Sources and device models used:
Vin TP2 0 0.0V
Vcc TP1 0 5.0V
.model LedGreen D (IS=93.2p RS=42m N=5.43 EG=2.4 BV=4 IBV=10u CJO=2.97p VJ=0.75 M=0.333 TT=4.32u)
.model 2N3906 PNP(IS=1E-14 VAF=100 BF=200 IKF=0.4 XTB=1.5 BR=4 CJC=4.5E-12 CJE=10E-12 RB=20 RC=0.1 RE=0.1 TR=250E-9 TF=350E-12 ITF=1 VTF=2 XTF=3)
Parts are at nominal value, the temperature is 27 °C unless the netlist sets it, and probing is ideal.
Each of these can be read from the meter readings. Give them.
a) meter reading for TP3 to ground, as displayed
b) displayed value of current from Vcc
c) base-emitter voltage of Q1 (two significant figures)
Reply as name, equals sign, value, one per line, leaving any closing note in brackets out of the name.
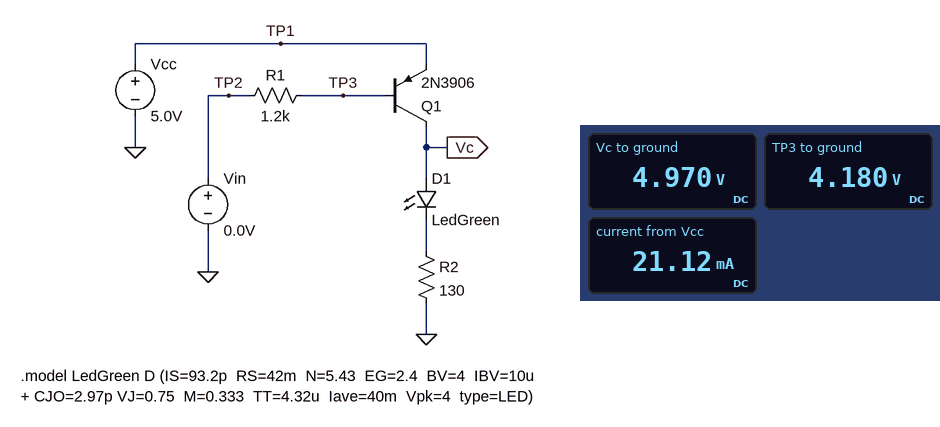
meter reading for TP3 to ground, as displayed = 4.180 V
displayed value of current from Vcc = 21.12 mA
base-emitter voltage of Q1 = -820 mV
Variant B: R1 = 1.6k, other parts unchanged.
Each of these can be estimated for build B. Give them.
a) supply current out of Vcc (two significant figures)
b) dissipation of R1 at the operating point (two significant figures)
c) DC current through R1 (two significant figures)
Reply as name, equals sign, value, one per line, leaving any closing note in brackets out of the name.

supply current out of Vcc = 20 mA
dissipation of R1 at the operating point = 11 mW
DC current through R1 = 2.6 mA
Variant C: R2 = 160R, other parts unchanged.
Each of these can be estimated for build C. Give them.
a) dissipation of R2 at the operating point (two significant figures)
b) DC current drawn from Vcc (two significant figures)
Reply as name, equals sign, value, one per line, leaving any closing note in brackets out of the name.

dissipation of R2 at the operating point = 34 mW
DC current drawn from Vcc = 18 mA
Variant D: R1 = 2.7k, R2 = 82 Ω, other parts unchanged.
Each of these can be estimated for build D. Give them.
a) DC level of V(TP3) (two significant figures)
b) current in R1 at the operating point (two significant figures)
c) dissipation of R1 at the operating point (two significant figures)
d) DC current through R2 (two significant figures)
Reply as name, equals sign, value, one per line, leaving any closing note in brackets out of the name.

DC level of V(TP3) = 4.2 V
current in R1 at the operating point = 1.6 mA
dissipation of R1 at the operating point = 6.6 mW
DC current through R2 = 27 mA
